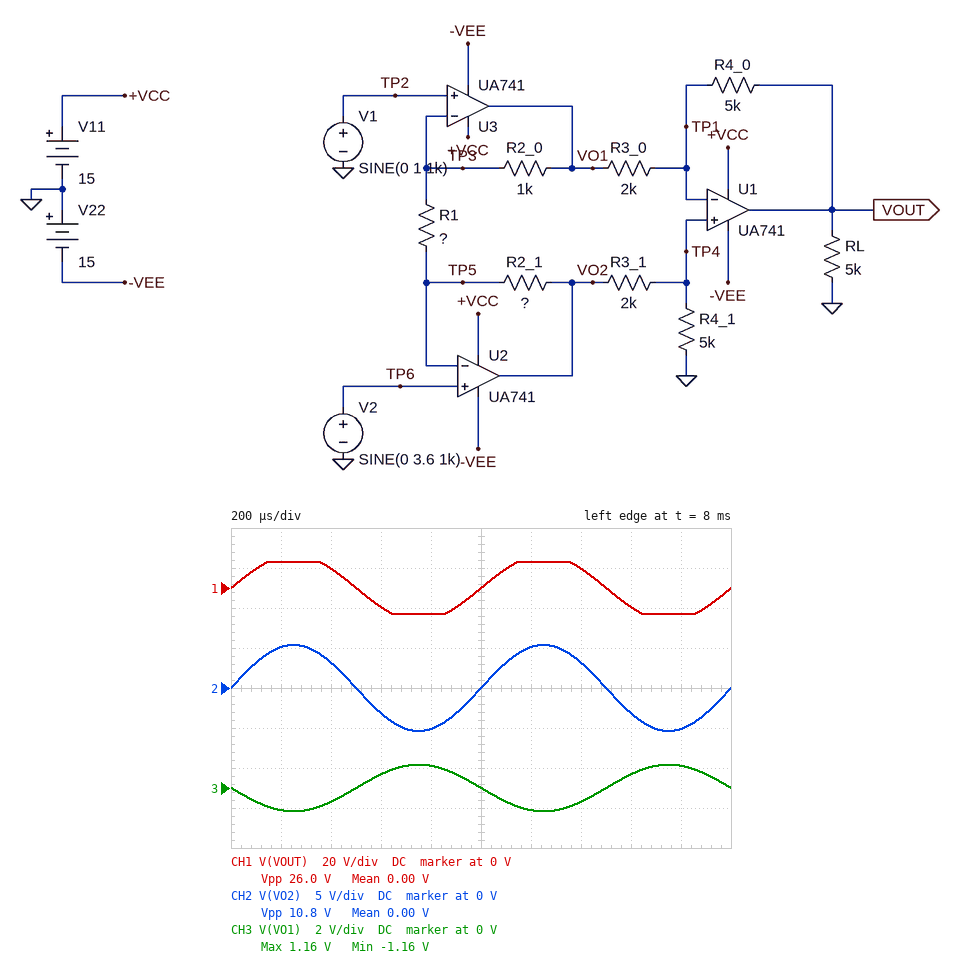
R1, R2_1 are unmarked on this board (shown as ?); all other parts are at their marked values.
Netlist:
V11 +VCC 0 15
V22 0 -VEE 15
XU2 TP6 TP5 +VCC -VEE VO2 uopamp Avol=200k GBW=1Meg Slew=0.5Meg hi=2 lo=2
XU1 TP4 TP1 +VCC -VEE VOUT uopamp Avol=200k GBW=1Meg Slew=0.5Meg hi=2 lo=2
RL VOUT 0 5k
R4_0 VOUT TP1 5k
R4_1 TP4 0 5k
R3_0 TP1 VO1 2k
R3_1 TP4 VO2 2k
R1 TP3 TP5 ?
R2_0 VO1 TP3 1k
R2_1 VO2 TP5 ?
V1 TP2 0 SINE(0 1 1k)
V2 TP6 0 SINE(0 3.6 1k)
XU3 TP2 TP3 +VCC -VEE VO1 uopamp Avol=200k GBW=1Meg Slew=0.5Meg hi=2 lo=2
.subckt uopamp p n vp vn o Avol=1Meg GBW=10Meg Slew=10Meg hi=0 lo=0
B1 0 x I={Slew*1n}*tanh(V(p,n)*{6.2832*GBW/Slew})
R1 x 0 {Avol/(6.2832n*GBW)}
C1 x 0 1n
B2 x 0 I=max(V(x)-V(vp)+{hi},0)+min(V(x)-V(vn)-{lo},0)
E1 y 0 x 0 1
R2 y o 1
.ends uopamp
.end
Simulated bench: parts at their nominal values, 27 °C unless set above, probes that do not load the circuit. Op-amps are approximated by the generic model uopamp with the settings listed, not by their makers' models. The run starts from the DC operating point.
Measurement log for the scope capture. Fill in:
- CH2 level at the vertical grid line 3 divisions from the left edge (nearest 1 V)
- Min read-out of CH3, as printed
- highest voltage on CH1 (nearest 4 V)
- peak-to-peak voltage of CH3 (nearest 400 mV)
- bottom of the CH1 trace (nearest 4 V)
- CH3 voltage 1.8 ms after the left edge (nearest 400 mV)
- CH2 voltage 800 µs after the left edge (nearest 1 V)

-3 V
-1.16 V
12 V
2.4 V
-12 V
1.2 V
-5 V
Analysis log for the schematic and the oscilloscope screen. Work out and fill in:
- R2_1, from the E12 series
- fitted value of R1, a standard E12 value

820 Ω
1.2 kΩ
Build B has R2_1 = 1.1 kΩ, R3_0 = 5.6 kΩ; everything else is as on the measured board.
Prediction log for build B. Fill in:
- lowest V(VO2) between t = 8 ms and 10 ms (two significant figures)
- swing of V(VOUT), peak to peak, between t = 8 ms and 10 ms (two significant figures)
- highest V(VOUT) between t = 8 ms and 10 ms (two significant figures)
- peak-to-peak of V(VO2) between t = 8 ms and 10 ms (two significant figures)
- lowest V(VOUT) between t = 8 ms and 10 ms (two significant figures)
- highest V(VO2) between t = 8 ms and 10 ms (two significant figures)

-6.0 V
18 V
9.1 V
12 V
-9.1 V
6.0 V
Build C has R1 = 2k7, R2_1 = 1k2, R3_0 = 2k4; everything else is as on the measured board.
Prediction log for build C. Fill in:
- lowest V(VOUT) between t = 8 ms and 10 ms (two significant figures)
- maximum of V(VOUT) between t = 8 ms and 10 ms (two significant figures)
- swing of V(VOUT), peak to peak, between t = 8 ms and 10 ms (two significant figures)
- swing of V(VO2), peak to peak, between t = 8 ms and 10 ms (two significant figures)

-10 V
10 V
21 V
9.5 V
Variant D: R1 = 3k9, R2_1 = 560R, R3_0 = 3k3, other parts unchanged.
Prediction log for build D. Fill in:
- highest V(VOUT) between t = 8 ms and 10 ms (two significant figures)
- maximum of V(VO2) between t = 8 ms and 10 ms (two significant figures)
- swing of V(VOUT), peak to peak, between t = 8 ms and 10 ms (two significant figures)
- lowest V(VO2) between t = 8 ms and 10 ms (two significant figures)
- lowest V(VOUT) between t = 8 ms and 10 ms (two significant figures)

6.6 V
4.0 V
13 V
-4.0 V
-6.6 V
